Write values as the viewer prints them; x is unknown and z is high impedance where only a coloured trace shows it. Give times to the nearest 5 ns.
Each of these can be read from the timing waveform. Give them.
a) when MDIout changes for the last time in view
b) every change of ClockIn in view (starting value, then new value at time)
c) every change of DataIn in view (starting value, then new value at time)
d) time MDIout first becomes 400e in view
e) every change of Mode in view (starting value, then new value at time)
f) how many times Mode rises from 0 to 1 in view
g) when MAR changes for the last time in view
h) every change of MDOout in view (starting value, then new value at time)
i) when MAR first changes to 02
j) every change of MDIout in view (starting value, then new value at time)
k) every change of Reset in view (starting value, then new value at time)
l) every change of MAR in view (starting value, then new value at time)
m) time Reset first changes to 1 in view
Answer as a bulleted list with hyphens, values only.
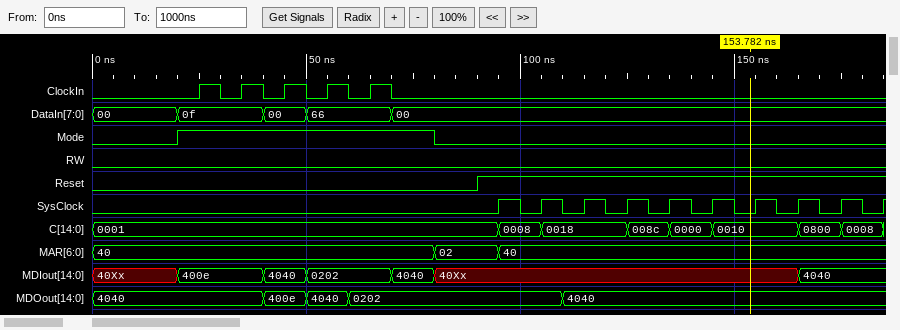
- 165 ns
- 0, 1 at 25 ns, 0 at 30 ns, 1 at 35 ns, 0 at 40 ns, 1 at 45 ns, 0 at 50 ns, 1 at 55 ns, 0 at 60 ns, 1 at 65 ns, 0 at 70 ns
- 00, 0f at 20 ns, 00 at 40 ns, 66 at 50 ns, 00 at 70 ns
- 20 ns
- 0, 1 at 20 ns, 0 at 80 ns
- 1
- 95 ns
- 4040, 400e at 40 ns, 4040 at 50 ns, 0202 at 60 ns, 4040 at 110 ns
- 80 ns
- 40Xx, 400e at 20 ns, 4040 at 40 ns, 0202 at 50 ns, 4040 at 70 ns, 40Xx at 80 ns, 4040 at 165 ns
- 0, 1 at 90 ns
- 40, 02 at 80 ns, 40 at 95 ns
- 90 ns
